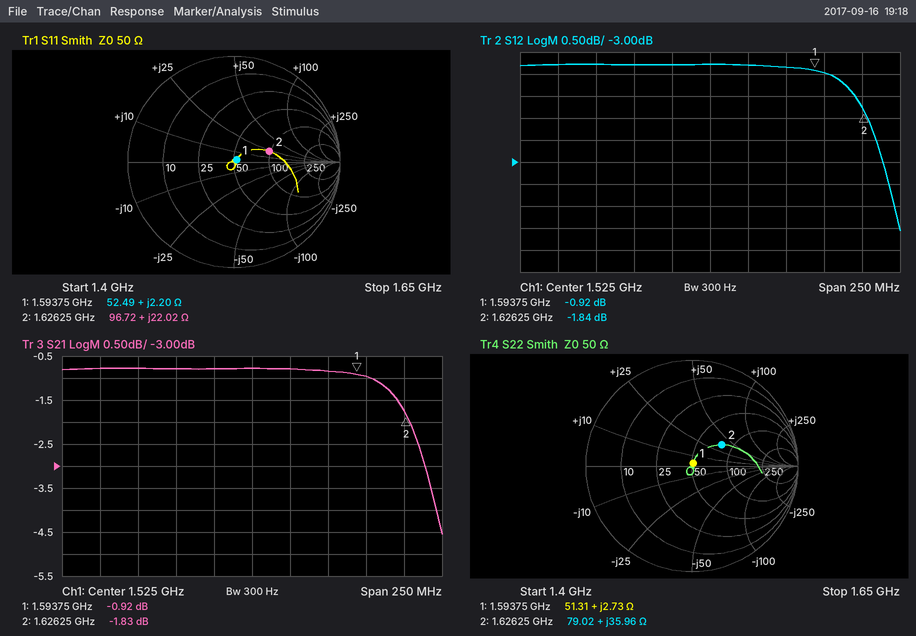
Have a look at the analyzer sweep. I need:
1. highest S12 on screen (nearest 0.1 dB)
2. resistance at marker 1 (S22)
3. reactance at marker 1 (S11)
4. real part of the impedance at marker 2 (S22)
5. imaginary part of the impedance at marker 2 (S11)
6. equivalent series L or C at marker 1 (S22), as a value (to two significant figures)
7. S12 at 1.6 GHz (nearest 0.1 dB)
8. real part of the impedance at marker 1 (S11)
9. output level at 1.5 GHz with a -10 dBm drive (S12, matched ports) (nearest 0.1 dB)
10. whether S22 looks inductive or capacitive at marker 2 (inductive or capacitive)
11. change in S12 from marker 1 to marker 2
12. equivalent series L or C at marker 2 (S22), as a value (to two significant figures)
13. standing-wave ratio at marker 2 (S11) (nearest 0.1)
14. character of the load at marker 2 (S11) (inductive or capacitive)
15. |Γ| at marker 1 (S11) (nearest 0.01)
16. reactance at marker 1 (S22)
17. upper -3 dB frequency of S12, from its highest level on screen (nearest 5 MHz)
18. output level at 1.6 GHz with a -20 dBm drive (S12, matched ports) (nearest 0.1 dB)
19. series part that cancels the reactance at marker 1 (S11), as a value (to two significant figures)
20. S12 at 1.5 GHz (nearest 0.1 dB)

-0.8 dB
51.31 Ω
+2.20 Ω
79.02 Ω
+22.02 Ω
270 pH
-1.0 dB
52.49 Ω
-10.8 dBm
inductive
-0.92 dB
3.5 nH
2.1
inductive
0.03
+2.73 Ω
1.645 GHz
-21.0 dBm
45 pF
-0.8 dB
